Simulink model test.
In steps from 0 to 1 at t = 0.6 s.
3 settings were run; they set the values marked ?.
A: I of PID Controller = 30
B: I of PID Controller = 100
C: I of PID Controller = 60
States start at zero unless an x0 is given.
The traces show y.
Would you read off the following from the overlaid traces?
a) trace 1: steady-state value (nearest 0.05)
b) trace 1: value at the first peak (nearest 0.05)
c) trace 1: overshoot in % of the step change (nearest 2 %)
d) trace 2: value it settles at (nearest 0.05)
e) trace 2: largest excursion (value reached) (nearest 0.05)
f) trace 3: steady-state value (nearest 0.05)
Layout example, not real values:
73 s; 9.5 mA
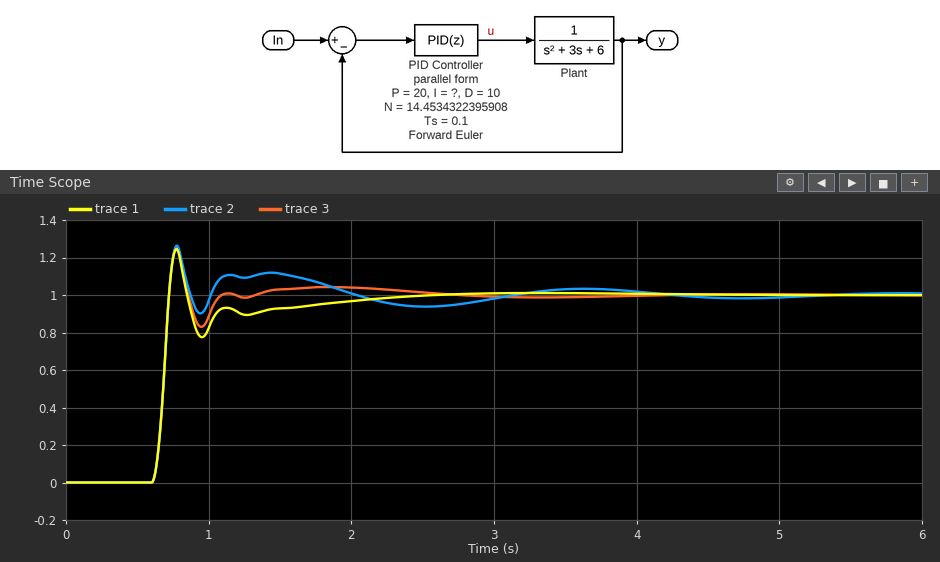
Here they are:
1.00; 1.25; 24 %; 1.00; 1.25; 1.00
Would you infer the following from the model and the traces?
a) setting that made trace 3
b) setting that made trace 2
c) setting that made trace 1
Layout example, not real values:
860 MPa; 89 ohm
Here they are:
C; B; A
